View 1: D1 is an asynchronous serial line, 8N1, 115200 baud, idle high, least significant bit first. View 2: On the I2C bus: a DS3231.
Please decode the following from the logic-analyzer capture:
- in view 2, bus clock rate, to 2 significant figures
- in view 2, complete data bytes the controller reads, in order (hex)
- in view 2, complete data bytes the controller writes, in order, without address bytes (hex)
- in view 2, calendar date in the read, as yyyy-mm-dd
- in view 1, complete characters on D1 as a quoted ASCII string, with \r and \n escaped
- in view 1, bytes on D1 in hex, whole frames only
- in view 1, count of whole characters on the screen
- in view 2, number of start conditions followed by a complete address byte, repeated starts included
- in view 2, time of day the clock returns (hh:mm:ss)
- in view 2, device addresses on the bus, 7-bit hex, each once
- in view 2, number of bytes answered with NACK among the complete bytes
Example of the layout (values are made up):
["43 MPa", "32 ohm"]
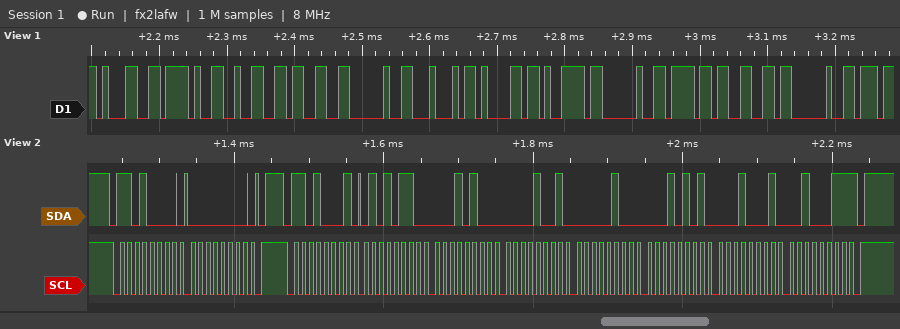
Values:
["100 kHz", "56 14 09 04 15 11 23", "00", "2023-11-15", "\"1/23 Day of \"", "31 2F 32 33 20 44 61 79 20 6F 66 20", "12", "2", "09:14:56", "0x68", "1"]
